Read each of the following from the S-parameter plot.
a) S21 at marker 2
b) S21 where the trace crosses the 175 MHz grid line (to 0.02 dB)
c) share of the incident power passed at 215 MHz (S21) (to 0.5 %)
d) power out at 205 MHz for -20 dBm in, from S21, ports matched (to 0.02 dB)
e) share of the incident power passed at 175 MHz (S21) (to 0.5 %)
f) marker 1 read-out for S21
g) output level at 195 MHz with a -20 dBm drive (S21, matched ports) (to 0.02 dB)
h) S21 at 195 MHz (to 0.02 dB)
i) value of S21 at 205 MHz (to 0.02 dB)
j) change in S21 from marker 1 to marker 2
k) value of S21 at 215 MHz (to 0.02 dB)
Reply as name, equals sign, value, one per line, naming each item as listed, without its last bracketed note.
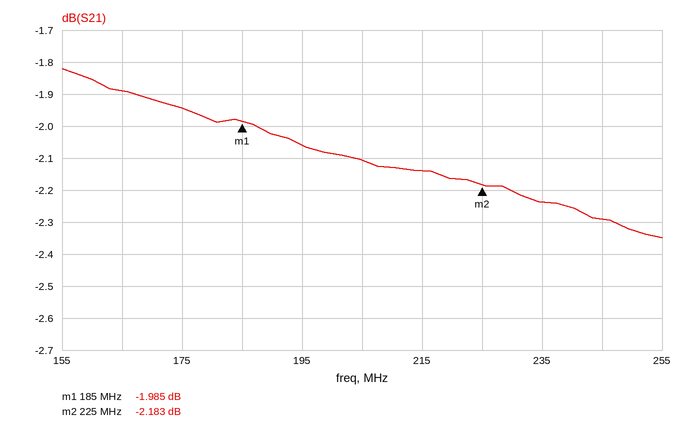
S21 at marker 2 = -2.183 dB
S21 where the trace crosses the 175 MHz grid line = -1.94 dB
share of the incident power passed at 215 MHz (S21) = 61.0 %
power out at 205 MHz for -20 dBm in, from S21, ports matched = -22.10 dBm
share of the incident power passed at 175 MHz (S21) = 64.0 %
marker 1 read-out for S21 = -1.985 dB
output level at 195 MHz with a -20 dBm drive (S21, matched ports) = -22.06 dBm
S21 at 195 MHz = -2.06 dB
value of S21 at 205 MHz = -2.10 dB
change in S21 from marker 1 to marker 2 = -0.198 dB
value of S21 at 215 MHz = -2.14 dB
